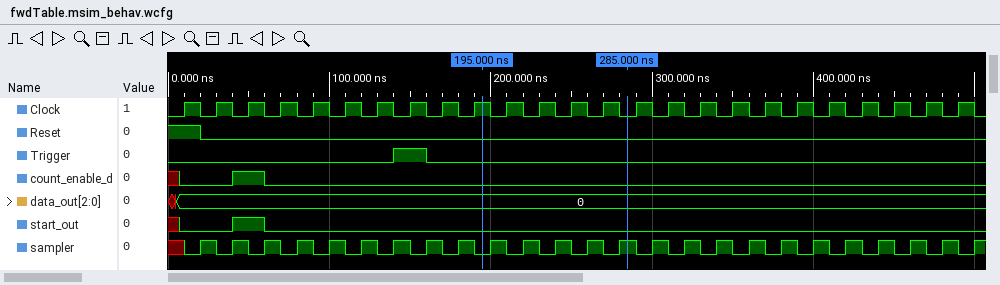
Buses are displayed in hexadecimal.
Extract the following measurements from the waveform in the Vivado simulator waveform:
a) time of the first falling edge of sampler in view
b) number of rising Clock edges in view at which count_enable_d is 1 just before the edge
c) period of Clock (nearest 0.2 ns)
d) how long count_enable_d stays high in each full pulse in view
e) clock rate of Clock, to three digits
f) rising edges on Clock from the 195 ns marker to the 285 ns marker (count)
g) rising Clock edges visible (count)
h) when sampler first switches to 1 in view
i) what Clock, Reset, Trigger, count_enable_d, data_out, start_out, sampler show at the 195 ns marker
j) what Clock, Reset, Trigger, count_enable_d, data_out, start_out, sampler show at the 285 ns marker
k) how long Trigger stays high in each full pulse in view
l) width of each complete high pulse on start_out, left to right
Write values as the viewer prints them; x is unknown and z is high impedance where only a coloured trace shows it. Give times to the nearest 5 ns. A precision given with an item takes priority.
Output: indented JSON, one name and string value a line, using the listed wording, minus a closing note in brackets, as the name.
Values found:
{
  "time of the first falling edge of sampler in view": "30 ns",
  "number of rising Clock edges in view at which count_enable_d is 1 just before the edge": "1",
  "period of Clock": "20 ns",
  "how long count_enable_d stays high in each full pulse in view": "20 ns",
  "clock rate of Clock, to three digits": "50.0 MHz",
  "rising edges on Clock from the 195 ns marker to the 285 ns marker": "4",
  "rising Clock edges visible": "25",
  "when sampler first switches to 1 in view": "20 ns",
  "what Clock, Reset, Trigger, count_enable_d, data_out, start_out, sampler show at the 195 ns marker": "Clock=1, Reset=0, Trigger=0, count_enable_d=0, data_out=0, start_out=0, sampler=0",
  "what Clock, Reset, Trigger, count_enable_d, data_out, start_out, sampler show at the 285 ns marker": "Clock=0, Reset=0, Trigger=0, count_enable_d=0, data_out=0, start_out=0, sampler=1",
  "how long Trigger stays high in each full pulse in view": "20 ns",
  "width of each complete high pulse on start_out, left to right": "20 ns"
}
